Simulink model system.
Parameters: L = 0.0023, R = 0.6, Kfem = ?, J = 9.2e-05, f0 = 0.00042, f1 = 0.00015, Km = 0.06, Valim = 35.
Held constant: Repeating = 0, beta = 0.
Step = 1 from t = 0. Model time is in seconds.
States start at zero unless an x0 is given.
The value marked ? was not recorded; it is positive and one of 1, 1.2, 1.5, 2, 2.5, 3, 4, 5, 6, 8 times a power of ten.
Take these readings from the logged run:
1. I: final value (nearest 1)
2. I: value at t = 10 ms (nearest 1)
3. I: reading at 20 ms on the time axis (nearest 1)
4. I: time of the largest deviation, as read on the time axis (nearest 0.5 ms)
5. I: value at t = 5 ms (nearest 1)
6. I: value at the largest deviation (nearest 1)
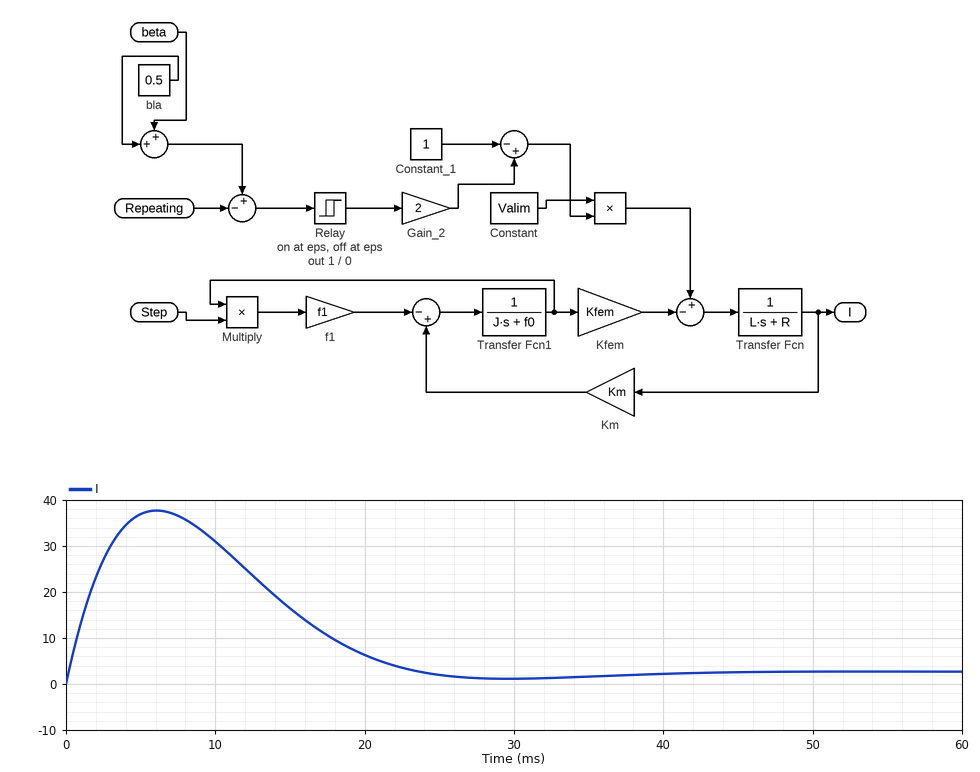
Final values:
3
31
6
6.0 ms
37
38
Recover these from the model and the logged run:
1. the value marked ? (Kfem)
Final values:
0.12
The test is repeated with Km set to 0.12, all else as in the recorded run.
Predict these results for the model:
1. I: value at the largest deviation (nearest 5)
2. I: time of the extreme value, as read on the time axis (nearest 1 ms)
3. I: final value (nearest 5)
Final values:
30
5 ms
0
